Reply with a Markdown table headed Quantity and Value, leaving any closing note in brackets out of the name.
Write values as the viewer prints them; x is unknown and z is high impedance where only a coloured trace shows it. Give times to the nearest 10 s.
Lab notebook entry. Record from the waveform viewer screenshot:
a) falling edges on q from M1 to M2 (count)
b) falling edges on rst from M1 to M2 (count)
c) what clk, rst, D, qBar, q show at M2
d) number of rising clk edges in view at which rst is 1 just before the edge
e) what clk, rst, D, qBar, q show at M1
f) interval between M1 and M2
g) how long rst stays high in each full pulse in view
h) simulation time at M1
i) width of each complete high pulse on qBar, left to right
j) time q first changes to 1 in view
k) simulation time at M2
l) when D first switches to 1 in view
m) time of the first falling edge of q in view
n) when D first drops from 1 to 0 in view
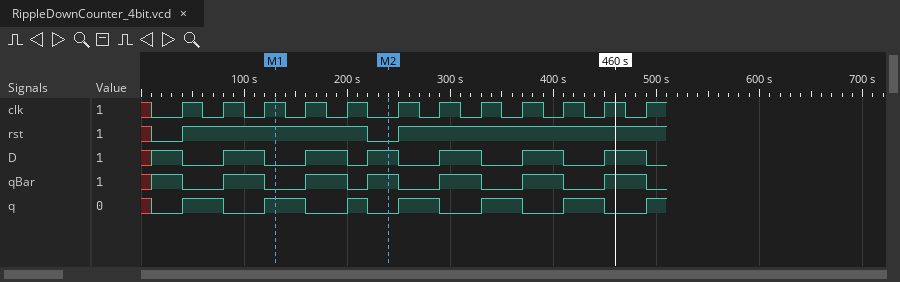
| Quantity | Value |
|---|---|
| falling edges on q from M1 to M2 | 2 |
| falling edges on rst from M1 to M2 | 1 |
| what clk, rst, D, qBar, q show at M2 | clk=0, rst=0, D=1, qBar=1, q=0 |
| number of rising clk edges in view at which rst is 1 just before the edge | 10 |
| what clk, rst, D, qBar, q show at M1 | clk=1, rst=1, D=0, qBar=0, q=1 |
| interval between M1 and M2 | 110 s |
| how long rst stays high in each full pulse in view | 180 s |
| simulation time at M1 | 130 s |
| width of each complete high pulse on qBar, left to right | 40 s, 40 s, 30 s, 40 s, 40 s, 40 s |
| time q first changes to 1 in view | 40 s |
| simulation time at M2 | 240 s |
| when D first switches to 1 in view | 10 s |
| time of the first falling edge of q in view | 80 s |
| when D first drops from 1 to 0 in view | 40 s |
